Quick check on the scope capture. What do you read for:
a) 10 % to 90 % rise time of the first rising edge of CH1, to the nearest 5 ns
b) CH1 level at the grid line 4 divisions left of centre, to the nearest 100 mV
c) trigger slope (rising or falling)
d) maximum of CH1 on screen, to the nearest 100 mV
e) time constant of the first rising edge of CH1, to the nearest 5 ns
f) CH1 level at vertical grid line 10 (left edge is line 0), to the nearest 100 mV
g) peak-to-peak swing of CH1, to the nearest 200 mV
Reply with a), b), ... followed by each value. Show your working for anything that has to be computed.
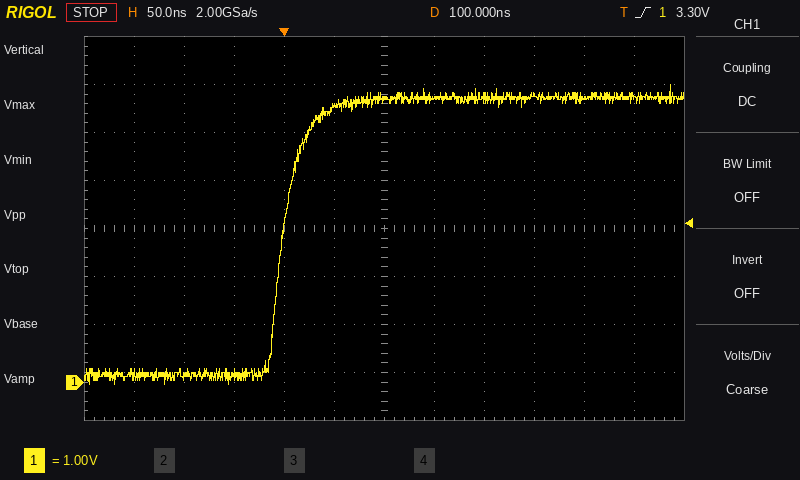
a) 40 ns
b) 100 mV
c) rising
d) 6.2 V
e) 40 ns / 2.2 ≈ 18.2 ns, so 20 ns to the nearest 5 ns
f) 5.9 V
g) 6.2 V
